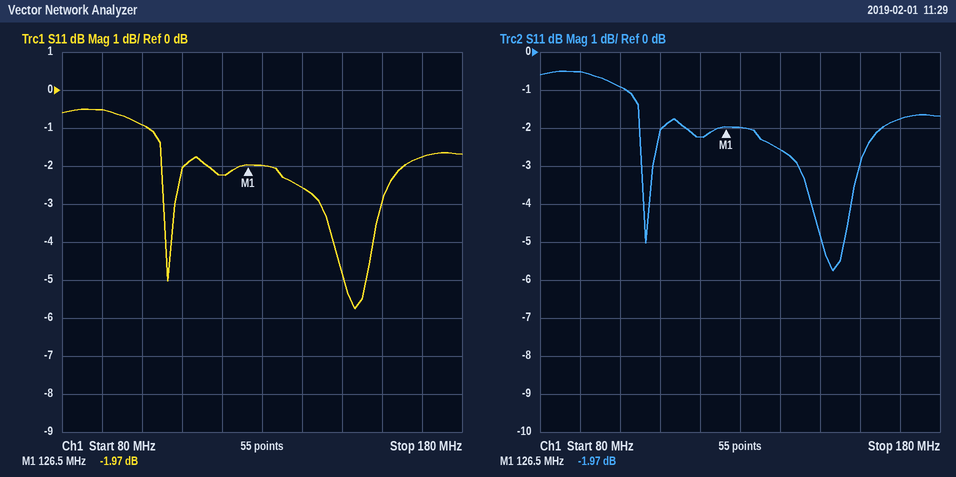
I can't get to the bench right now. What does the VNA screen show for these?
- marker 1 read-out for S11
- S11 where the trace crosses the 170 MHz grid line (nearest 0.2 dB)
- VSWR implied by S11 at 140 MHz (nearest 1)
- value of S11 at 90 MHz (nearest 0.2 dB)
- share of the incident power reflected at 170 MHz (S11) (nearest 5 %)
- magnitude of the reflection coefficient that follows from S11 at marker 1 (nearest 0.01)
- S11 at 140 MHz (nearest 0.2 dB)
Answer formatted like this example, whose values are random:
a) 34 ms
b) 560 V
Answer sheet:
a) -1.97 dB
b) -1.8 dB
c) 7
d) -0.6 dB
e) 65 %
f) 0.80
g) -2.6 dB
